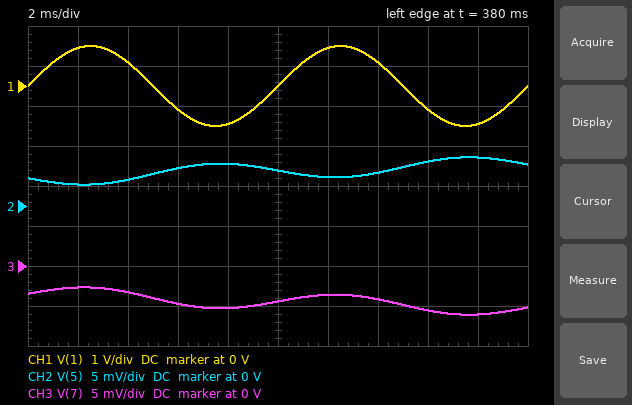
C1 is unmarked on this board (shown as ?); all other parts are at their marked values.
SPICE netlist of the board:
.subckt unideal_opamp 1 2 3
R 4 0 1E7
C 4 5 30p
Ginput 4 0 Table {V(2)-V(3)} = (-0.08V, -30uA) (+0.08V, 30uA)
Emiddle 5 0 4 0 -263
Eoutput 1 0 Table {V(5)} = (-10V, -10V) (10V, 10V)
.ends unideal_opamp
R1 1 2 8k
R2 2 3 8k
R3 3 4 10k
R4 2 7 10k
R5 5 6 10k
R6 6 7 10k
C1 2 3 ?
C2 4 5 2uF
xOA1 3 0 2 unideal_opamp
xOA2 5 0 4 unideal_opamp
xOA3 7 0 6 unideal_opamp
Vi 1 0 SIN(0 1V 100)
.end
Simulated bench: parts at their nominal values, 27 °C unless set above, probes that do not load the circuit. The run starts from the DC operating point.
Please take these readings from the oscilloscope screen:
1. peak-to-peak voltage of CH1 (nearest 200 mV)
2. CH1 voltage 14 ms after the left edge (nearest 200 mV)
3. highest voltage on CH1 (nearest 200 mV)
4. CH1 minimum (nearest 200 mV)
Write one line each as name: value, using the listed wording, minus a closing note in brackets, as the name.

peak-to-peak voltage of CH1: 2.0 V
CH1 voltage 14 ms after the left edge: 600 mV
highest voltage on CH1: 1.0 V
CH1 minimum: -1.0 V
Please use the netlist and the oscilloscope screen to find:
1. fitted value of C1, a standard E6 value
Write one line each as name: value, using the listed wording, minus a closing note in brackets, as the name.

fitted value of C1, a standard E6 value: 15 µF
